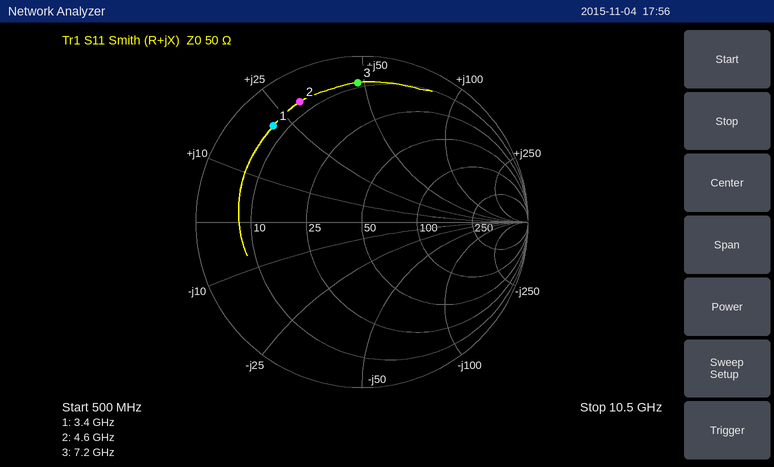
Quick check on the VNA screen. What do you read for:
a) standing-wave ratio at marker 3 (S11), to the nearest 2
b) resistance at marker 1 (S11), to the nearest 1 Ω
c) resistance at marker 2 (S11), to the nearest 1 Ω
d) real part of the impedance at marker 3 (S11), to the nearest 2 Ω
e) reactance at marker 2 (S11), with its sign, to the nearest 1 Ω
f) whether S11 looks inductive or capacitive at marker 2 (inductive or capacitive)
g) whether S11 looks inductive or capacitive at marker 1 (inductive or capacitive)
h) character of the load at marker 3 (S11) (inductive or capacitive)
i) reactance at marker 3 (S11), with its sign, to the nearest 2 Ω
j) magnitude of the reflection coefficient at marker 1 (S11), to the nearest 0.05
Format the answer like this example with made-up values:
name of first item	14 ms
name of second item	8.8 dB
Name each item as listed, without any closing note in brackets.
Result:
standing-wave ratio at marker 3 (S11), to the nearest 2	12
resistance at marker 1 (S11), to the nearest 1 Ω	7 Ω
resistance at marker 2 (S11), to the nearest 1 Ω	7 Ω
real part of the impedance at marker 3 (S11), to the nearest 2 Ω	8 Ω
reactance at marker 2 (S11), with its sign, to the nearest 1 Ω	+30 Ω
whether S11 looks inductive or capacitive at marker 2	inductive
whether S11 looks inductive or capacitive at marker 1	inductive
character of the load at marker 3 (S11)	inductive
reactance at marker 3 (S11), with its sign, to the nearest 2 Ω	+48 Ω
magnitude of the reflection coefficient at marker 1 (S11), to the nearest 0.05	0.80
